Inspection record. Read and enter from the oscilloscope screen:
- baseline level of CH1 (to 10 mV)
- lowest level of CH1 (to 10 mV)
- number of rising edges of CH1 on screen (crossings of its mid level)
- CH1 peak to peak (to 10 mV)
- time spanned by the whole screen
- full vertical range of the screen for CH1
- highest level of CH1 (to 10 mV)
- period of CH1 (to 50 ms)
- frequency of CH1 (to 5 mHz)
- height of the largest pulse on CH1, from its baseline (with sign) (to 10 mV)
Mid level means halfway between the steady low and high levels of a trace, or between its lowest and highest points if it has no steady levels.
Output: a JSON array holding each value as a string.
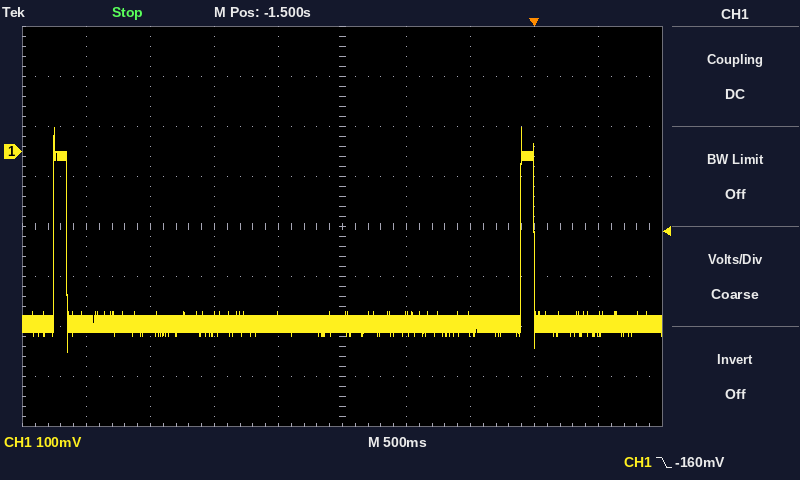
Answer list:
["-340 mV", "-400 mV", "2", "450 mV", "5 s", "800 mV", "50 mV", "3.65 s", "275 mHz", "+390 mV"]
